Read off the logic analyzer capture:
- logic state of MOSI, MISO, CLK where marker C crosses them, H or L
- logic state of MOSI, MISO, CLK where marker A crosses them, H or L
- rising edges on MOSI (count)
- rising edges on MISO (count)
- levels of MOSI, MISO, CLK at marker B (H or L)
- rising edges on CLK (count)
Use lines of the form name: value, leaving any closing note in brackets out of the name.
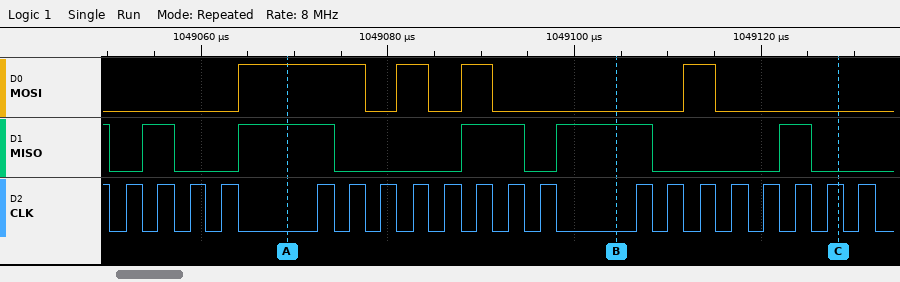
logic state of MOSI, MISO, CLK where marker C crosses them, H or L: MOSI=L, MISO=L, CLK=H
logic state of MOSI, MISO, CLK where marker A crosses them, H or L: MOSI=H, MISO=H, CLK=L
rising edges on MOSI: 4
rising edges on MISO: 5
levels of MOSI, MISO, CLK at marker B: MOSI=L, MISO=H, CLK=L
rising edges on CLK: 20
